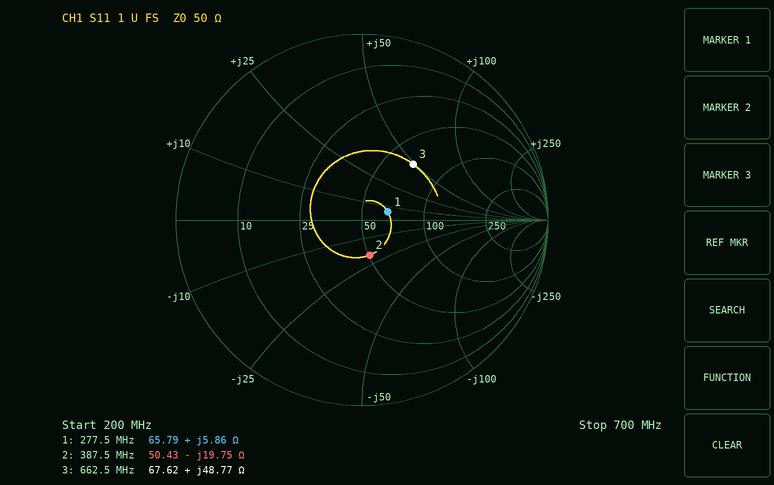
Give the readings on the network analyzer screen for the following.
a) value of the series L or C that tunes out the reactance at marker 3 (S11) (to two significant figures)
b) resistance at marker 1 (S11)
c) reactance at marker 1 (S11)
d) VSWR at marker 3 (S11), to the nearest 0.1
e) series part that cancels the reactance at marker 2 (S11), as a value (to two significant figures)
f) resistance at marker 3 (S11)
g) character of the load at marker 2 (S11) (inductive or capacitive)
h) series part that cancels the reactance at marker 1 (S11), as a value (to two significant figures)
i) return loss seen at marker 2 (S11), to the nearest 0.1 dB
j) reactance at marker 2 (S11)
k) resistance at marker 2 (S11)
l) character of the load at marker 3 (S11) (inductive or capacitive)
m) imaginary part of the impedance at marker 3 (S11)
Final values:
4.9 pF
65.79 Ω
+5.86 Ω
2.4
8.1 nH
67.62 Ω
capacitive
98 pF
14.3 dB
-19.75 Ω
50.43 Ω
inductive
+48.77 Ω
